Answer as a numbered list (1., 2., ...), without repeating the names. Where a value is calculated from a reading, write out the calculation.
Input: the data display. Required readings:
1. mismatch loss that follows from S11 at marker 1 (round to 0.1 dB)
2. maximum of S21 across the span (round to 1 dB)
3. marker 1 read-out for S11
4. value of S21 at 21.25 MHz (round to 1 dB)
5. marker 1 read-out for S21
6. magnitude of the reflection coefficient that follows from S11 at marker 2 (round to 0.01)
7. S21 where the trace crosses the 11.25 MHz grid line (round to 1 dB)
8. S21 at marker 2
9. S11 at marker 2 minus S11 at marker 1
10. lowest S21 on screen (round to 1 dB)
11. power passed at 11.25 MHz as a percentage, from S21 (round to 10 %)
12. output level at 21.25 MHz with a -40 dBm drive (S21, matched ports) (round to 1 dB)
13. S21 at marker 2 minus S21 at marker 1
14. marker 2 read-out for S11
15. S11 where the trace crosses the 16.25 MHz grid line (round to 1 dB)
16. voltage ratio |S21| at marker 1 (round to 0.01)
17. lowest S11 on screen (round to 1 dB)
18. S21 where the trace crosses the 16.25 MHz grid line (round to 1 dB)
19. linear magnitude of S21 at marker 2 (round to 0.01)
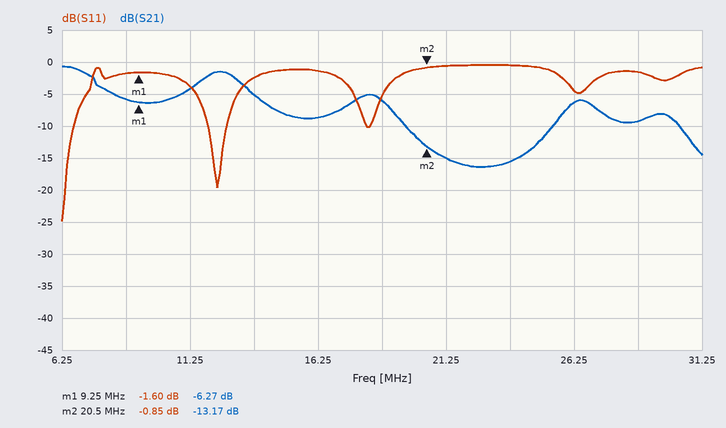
1. −10 log10(1 − 10^(-1.6/10)) ≈ 5.1 dB
2. -1 dB
3. -1.60 dB
4. -15 dB
5. -6.27 dB
6. 10^(-0.85/20) ≈ 0.91
7. -4 dB
8. -13.17 dB
9. -0.85 − (-1.6) = 0.75 dB
10. -16 dB
11. 10^(-4/10) ≈ 40 %
12. -40 dBm + (-15 dB) = -55 dBm
13. -13.17 − (-6.27) = -6.90 dB
14. -0.85 dB
15. -1 dB
16. 10^(-6.27/20) ≈ 0.49
17. -25 dB
18. -9 dB
19. 10^(-13.17/20) ≈ 0.22
